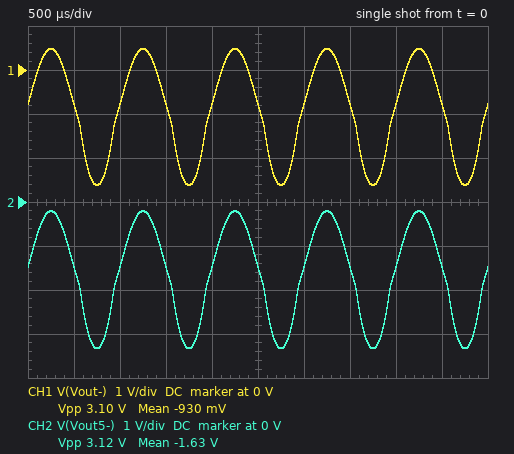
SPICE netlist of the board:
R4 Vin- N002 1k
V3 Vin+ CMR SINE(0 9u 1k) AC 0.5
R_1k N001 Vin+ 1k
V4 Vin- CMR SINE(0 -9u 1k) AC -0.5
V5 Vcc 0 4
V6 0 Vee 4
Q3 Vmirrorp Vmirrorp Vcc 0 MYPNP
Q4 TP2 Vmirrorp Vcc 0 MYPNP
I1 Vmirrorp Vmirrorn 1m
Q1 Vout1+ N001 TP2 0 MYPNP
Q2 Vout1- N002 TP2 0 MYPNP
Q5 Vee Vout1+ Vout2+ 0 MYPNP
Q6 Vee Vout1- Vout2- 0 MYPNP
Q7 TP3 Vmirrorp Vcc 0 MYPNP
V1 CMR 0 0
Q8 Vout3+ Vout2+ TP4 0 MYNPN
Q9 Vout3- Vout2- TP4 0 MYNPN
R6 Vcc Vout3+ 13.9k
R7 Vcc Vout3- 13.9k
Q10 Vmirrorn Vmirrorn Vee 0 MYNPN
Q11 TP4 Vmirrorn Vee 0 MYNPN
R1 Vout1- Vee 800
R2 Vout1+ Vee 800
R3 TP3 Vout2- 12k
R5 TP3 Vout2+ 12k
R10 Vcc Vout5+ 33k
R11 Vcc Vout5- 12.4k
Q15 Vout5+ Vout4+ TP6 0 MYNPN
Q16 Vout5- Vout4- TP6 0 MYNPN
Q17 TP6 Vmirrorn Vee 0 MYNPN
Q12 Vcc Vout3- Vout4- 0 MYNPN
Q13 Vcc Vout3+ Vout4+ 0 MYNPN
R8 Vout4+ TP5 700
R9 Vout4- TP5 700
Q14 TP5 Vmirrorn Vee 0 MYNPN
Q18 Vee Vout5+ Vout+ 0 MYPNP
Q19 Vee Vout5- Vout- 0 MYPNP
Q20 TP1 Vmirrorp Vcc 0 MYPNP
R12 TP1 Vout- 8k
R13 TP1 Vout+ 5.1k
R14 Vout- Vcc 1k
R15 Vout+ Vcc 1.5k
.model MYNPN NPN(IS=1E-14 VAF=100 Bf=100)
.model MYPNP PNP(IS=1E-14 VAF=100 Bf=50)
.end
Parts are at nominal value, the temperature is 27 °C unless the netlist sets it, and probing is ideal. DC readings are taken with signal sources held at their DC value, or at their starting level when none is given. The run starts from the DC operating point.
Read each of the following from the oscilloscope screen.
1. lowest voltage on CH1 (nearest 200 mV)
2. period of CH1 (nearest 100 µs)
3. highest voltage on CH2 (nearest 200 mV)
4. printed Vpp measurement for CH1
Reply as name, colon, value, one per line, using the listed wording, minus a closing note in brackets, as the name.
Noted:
lowest voltage on CH1: -2.6 V
period of CH1: 1.0 ms
highest voltage on CH2: -200 mV
printed Vpp measurement for CH1: 3.10 V
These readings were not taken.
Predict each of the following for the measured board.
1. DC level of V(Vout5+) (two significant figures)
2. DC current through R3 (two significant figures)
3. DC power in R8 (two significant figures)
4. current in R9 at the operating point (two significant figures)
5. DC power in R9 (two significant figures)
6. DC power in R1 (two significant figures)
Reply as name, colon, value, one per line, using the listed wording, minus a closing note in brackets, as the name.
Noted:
DC level of V(Vout5+): -3.8 V
DC current through R3: 470 µA
DC power in R8: 160 µW
current in R9 at the operating point: 480 µA
DC power in R9: 160 µW
DC power in R1: 180 µW
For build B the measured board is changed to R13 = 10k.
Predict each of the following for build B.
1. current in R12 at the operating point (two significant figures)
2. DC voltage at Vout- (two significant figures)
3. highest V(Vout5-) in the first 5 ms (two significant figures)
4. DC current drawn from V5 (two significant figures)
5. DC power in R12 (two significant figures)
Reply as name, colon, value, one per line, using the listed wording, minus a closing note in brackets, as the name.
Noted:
current in R12 at the operating point: 390 µA
DC voltage at Vout-: -770 mV
highest V(Vout5-) in the first 5 ms: -190 mV
DC current drawn from V5: 16 mA
DC power in R12: 1.2 mW
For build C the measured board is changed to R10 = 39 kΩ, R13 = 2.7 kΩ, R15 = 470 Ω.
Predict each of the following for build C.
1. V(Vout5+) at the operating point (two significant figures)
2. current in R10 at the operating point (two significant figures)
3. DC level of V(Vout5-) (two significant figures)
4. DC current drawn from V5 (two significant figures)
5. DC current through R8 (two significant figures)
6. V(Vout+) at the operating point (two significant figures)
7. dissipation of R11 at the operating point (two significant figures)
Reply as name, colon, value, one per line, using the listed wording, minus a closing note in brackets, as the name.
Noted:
V(Vout5+) at the operating point: -3.0 V
current in R10 at the operating point: 180 µA
DC level of V(Vout5-): -810 mV
DC current drawn from V5: 24 mA
DC current through R8: 480 µA
V(Vout+) at the operating point: -2.3 V
dissipation of R11 at the operating point: 1.9 mW
